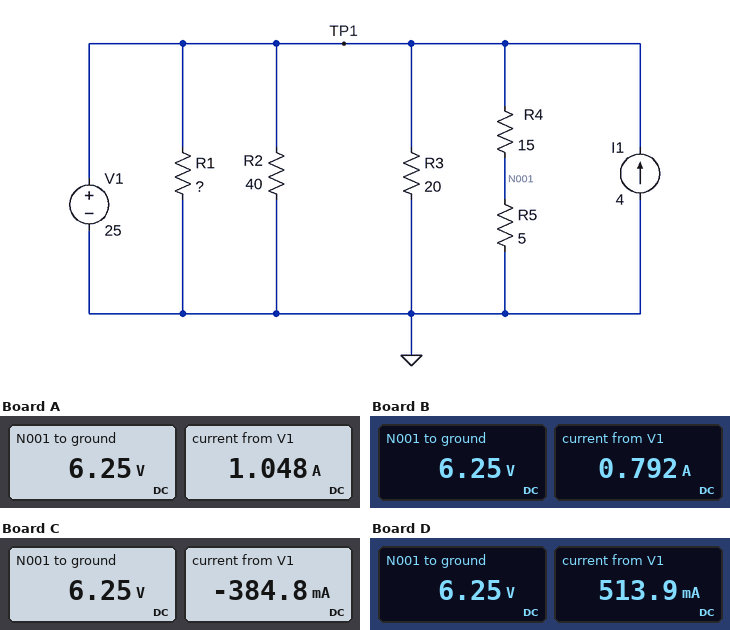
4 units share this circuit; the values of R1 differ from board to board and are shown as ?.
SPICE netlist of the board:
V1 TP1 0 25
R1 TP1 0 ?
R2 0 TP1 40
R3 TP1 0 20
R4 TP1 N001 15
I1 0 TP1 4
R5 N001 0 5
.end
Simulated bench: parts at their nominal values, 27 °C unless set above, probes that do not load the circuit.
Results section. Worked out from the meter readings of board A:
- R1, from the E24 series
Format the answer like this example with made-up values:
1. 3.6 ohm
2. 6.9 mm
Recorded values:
1. 13 Ω
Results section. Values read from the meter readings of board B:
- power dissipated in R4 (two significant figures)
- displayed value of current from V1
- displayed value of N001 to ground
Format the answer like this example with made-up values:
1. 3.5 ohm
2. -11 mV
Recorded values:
1. 23 W
2. 0.792 A
3. 6.25 V
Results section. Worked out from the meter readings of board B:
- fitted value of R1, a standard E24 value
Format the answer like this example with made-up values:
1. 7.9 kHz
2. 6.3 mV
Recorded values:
1. 15 Ω
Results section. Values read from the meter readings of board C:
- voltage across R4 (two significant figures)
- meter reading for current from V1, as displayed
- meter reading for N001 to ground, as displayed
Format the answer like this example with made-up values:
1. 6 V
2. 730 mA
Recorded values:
1. 19 V
2. -384.8 mA
3. 6.25 V
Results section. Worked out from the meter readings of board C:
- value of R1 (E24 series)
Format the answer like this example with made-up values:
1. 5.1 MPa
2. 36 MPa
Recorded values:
1. 51 Ω
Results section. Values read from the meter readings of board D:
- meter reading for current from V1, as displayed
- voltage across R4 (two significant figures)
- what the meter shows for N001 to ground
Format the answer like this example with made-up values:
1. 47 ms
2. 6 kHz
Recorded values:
1. 513.9 mA
2. 19 V
3. 6.25 V
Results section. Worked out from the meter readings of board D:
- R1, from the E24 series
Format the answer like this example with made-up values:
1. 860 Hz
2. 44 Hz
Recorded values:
1. 18 Ω
